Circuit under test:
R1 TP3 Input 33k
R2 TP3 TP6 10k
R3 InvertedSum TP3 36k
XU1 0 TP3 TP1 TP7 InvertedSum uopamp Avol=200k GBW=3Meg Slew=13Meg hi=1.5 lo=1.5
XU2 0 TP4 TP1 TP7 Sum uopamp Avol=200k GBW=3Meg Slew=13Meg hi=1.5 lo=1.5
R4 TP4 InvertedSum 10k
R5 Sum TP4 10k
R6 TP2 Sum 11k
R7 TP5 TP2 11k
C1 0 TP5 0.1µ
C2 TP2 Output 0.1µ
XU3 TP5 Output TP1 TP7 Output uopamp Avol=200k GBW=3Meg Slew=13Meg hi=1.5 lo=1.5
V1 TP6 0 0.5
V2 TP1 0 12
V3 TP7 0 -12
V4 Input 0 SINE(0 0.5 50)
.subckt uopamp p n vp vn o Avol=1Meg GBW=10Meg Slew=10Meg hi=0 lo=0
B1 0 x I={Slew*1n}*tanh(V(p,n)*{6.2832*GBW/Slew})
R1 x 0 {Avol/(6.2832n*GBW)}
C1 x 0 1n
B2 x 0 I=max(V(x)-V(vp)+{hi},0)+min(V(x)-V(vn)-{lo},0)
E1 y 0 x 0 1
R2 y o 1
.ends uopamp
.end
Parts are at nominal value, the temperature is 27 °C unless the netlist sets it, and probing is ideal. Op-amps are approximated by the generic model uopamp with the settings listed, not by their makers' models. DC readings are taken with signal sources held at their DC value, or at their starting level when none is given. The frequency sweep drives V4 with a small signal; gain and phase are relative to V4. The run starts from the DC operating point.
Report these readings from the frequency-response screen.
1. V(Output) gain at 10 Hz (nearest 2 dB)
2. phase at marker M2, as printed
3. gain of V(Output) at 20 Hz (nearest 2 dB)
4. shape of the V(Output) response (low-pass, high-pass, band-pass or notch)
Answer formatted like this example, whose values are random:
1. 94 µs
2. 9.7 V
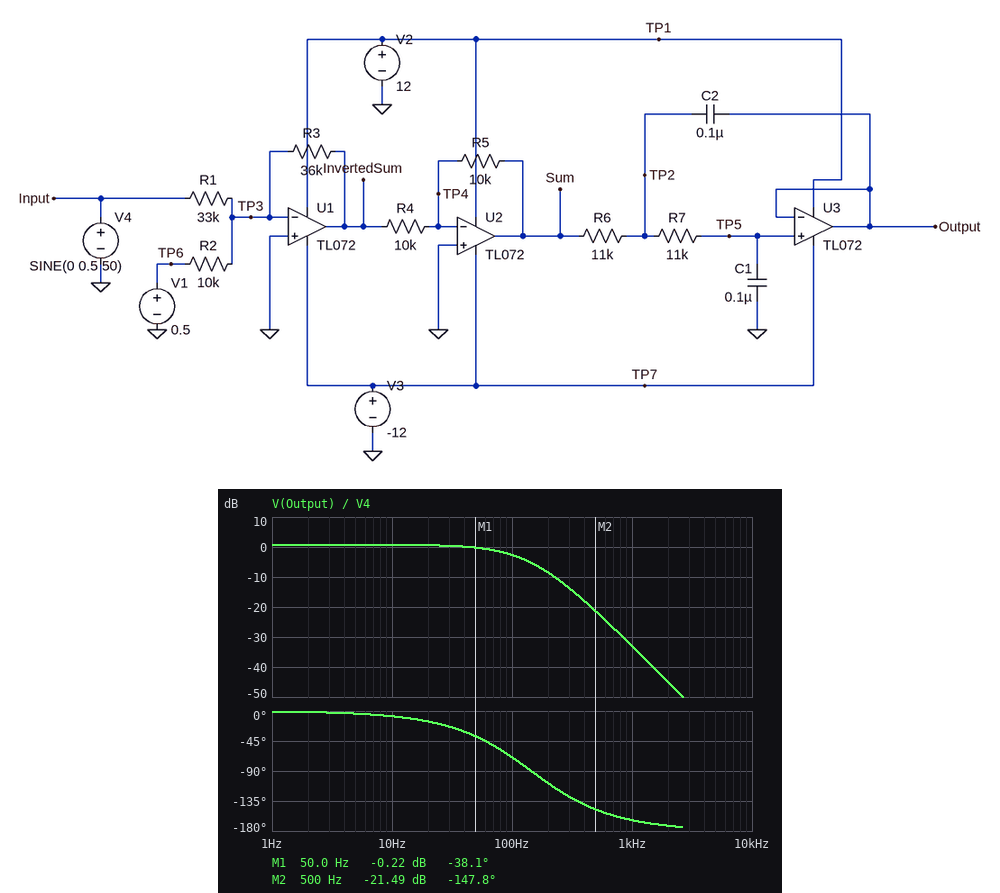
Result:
1. 0 dB
2. -147.8 deg
3. 0 dB
4. low-pass
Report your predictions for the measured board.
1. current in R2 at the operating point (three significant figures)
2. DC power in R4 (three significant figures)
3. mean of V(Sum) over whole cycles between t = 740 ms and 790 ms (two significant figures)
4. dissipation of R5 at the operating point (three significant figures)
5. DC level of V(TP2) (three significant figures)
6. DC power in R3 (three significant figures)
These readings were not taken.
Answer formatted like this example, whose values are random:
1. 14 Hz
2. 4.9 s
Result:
1. 50.0 µA
2. 324 µW
3. 1.8 V
4. 324 µW
5. 1.80 V
6. 90.0 µW
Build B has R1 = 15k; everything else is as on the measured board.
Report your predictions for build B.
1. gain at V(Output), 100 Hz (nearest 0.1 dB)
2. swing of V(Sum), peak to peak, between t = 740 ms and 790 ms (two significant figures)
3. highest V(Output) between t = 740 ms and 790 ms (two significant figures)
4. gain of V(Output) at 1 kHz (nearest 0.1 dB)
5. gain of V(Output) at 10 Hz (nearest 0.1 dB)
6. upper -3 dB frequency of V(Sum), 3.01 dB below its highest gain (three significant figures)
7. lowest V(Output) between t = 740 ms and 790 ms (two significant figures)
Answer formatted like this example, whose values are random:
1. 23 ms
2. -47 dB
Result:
1. 4.2 dB
2. 2.4 V
3. 2.9 V
4. -26.2 dB
5. 7.6 dB
6. 399 kHz
7. 730 mV
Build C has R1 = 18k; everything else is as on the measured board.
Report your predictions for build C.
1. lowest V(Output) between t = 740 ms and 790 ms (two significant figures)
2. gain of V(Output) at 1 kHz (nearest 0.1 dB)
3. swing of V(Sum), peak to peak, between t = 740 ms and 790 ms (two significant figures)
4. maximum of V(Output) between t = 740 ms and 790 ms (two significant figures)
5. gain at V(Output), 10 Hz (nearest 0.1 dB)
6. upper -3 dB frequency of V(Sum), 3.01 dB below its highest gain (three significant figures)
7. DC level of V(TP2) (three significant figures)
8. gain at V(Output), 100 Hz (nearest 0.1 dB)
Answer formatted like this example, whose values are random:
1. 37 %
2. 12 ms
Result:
1. 910 mV
2. -27.7 dB
3. 2.0 V
4. 2.7 V
5. 6.0 dB
6. 420 kHz
7. 1.80 V
8. 2.6 dB
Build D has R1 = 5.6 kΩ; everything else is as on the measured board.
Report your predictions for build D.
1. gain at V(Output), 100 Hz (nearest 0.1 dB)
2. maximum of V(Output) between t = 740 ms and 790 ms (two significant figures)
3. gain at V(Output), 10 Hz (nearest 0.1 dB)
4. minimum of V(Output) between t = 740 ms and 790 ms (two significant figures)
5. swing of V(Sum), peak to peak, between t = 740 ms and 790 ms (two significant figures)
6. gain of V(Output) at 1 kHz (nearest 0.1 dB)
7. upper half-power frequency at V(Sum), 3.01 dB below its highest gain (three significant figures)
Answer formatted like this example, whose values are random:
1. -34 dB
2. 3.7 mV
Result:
1. 12.8 dB
2. 4.7 V
3. 16.1 dB
4. -1.1 V
5. 6.4 V
6. -17.6 dB
7. 264 kHz
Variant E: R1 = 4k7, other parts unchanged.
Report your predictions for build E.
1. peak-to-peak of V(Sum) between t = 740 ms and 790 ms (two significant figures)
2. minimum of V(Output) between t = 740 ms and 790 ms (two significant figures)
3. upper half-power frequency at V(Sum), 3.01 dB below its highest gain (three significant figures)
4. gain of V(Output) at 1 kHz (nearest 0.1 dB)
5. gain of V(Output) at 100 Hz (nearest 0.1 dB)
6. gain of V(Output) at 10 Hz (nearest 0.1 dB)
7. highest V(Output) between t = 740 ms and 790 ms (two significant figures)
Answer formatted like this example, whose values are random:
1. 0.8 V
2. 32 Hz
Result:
1. 7.7 V
2. -1.6 V
3. 239 kHz
4. -16.1 dB
5. 14.3 dB
6. 17.6 dB
7. 5.2 V
